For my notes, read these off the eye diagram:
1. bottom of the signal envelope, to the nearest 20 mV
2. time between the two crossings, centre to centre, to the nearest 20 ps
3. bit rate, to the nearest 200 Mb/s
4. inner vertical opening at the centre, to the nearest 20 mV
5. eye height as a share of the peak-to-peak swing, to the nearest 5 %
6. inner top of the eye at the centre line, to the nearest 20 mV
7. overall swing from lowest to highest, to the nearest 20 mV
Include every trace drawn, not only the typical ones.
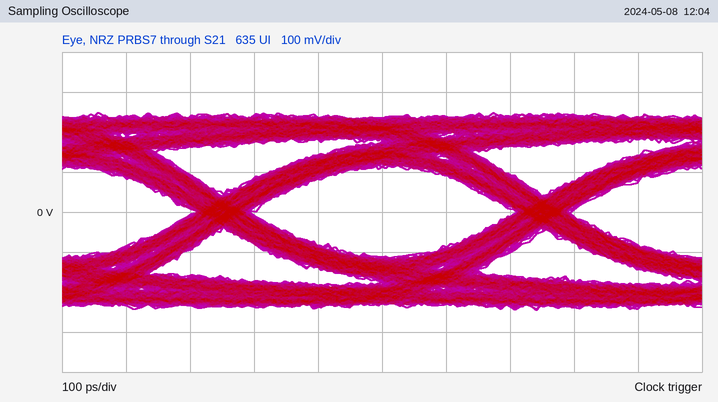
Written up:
-240 mV
500 ps
2.0 Gb/s
220 mV
45 %
120 mV
500 mV
